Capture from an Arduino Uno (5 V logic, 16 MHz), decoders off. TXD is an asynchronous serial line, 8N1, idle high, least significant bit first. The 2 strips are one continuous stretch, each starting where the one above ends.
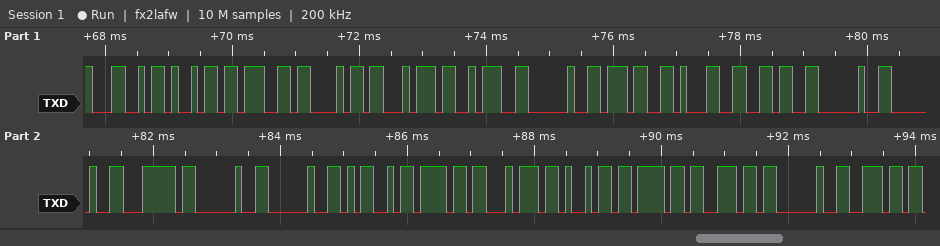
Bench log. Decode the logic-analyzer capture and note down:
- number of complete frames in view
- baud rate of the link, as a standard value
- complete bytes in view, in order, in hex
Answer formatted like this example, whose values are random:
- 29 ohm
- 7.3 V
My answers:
- 23
- 9600 baud
- 4C 69 67 68 74 3A 20 37 31 36 20 20 7C 20 20 4D 6F 74 69 6F 6E 20 6E
